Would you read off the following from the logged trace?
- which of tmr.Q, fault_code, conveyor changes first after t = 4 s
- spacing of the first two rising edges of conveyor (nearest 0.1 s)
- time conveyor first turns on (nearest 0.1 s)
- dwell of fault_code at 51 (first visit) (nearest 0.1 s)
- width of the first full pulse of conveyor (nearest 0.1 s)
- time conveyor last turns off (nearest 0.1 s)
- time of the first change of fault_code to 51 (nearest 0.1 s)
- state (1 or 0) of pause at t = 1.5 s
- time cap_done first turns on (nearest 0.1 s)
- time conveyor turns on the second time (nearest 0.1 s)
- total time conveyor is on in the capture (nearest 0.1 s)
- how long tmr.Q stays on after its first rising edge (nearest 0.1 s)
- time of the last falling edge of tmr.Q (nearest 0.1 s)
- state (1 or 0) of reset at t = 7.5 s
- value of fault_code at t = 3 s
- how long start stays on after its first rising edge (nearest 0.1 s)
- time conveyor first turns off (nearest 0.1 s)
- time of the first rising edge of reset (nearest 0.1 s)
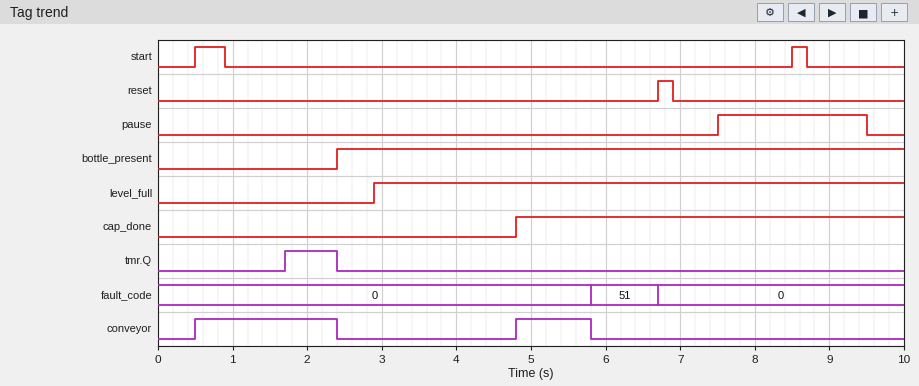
conveyor
4.3 s
0.5 s
0.9 s
1.9 s
5.8 s
5.8 s
0
4.8 s
4.8 s
2.9 s
0.7 s
2.4 s
0
0
0.4 s
2.4 s
6.7 s
